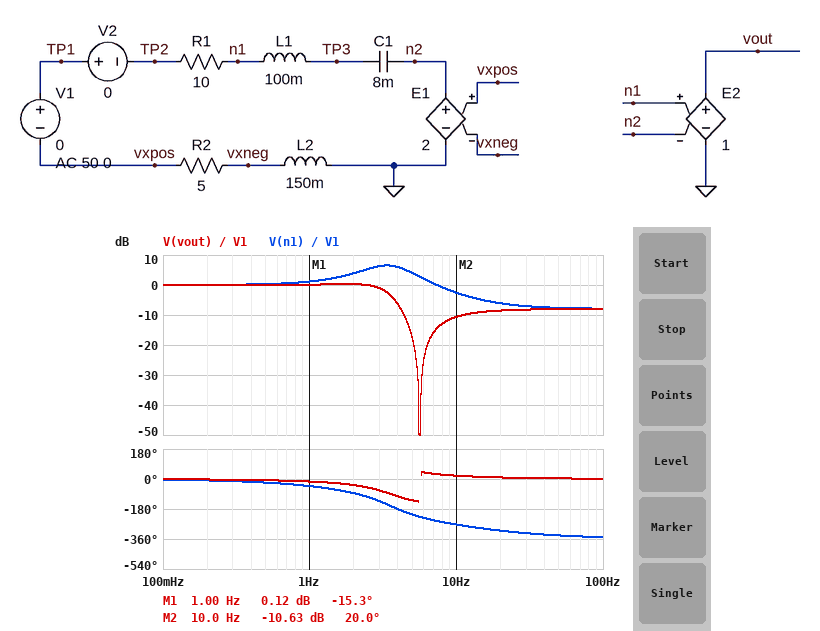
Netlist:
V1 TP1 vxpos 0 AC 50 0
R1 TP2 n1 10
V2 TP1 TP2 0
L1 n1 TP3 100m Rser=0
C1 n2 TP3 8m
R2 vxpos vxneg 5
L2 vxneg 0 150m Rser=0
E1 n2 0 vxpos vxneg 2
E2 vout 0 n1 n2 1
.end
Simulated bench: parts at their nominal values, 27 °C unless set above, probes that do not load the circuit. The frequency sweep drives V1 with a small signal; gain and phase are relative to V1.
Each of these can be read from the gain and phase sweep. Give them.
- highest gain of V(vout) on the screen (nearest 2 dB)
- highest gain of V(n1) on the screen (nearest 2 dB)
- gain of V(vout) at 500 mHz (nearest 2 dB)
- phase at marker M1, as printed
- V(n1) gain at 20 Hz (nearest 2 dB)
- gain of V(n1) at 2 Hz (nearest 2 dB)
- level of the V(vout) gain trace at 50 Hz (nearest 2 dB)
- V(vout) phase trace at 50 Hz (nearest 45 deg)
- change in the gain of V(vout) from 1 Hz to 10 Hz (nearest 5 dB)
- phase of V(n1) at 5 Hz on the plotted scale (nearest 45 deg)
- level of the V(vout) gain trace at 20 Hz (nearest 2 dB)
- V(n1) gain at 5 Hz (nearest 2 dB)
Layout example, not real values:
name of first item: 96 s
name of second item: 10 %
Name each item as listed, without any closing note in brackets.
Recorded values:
highest gain of V(vout) on the screen: 0 dB
highest gain of V(n1) on the screen: 6 dB
gain of V(vout) at 500 mHz: 0 dB
phase at marker M1, as printed: -15.3 deg
V(n1) gain at 20 Hz: -6 dB
gain of V(n1) at 2 Hz: 4 dB
level of the V(vout) gain trace at 50 Hz: -8 dB
V(vout) phase trace at 50 Hz: 0 deg
change in the gain of V(vout) from 1 Hz to 10 Hz: -10 dB
phase of V(n1) at 5 Hz on the plotted scale: -225 deg
level of the V(vout) gain trace at 20 Hz: -8 dB
V(n1) gain at 5 Hz: 4 dB
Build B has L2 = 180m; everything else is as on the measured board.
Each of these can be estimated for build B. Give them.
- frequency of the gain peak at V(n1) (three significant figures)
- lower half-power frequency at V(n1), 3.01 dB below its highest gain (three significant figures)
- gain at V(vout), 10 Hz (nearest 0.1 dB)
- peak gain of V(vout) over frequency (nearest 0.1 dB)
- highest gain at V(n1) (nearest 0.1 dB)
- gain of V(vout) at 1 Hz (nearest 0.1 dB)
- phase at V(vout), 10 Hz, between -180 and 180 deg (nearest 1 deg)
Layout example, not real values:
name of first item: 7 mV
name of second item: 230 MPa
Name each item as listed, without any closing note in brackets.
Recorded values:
frequency of the gain peak at V(n1): 3.19 Hz
lower half-power frequency at V(n1), 3.01 dB below its highest gain: 1.83 Hz
gain at V(vout), 10 Hz: -11.6 dB
peak gain of V(vout) over frequency: 0.6 dB
highest gain at V(n1): 6.7 dB
gain of V(vout) at 1 Hz: 0.2 dB
phase at V(vout), 10 Hz, between -180 and 180 deg: 18 deg
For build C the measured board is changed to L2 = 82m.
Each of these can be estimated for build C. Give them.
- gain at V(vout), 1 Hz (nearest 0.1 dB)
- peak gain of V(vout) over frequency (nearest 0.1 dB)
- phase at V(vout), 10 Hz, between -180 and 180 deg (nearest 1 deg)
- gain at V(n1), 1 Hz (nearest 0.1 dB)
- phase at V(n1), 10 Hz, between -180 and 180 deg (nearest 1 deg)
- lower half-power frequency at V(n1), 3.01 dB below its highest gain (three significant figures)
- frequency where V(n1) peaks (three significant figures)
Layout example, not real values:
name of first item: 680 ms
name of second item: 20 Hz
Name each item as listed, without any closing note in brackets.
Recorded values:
gain at V(vout), 1 Hz: -0.1 dB
peak gain of V(vout) over frequency: 0 dB
phase at V(vout), 10 Hz, between -180 and 180 deg: 28 deg
gain at V(n1), 1 Hz: 1.0 dB
phase at V(n1), 10 Hz, between -180 and 180 deg: 95 deg
lower half-power frequency at V(n1), 3.01 dB below its highest gain: 2.01 Hz
frequency where V(n1) peaks: 3.97 Hz
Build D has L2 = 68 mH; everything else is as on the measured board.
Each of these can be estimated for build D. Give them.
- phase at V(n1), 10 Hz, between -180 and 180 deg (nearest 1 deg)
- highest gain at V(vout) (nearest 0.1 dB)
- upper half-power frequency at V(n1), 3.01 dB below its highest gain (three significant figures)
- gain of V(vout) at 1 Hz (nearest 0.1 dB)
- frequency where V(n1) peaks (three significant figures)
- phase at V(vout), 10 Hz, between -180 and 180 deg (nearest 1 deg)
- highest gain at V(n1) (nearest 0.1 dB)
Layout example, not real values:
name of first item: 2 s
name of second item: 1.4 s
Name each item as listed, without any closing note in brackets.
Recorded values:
phase at V(n1), 10 Hz, between -180 and 180 deg: 97 deg
highest gain at V(vout): 0 dB
upper half-power frequency at V(n1), 3.01 dB below its highest gain: 7.29 Hz
gain of V(vout) at 1 Hz: -0.1 dB
frequency where V(n1) peaks: 4.14 Hz
phase at V(vout), 10 Hz, between -180 and 180 deg: 30 deg
highest gain at V(n1): 6.2 dB
